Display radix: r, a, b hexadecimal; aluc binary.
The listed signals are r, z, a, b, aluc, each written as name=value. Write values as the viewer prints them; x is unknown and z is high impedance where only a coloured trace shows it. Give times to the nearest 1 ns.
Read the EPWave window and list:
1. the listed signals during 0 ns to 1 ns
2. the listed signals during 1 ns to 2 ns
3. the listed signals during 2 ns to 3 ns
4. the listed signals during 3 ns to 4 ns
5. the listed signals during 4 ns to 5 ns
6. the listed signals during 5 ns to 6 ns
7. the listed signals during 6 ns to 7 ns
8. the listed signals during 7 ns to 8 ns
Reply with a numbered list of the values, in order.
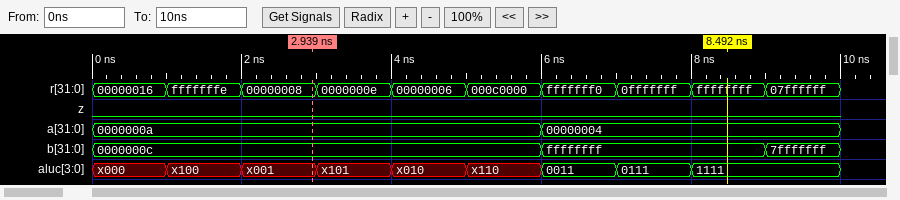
1. r=00000016, z=0, a=0000000a, b=0000000c, aluc=x000
2. r=fffffffe, z=0, a=0000000a, b=0000000c, aluc=x100
3. r=00000008, z=0, a=0000000a, b=0000000c, aluc=x001
4. r=0000000e, z=0, a=0000000a, b=0000000c, aluc=x101
5. r=00000006, z=0, a=0000000a, b=0000000c, aluc=x010
6. r=000c0000, z=0, a=0000000a, b=0000000c, aluc=x110
7. r=fffffff0, z=0, a=00000004, b=ffffffff, aluc=0011
8. r=0fffffff, z=0, a=00000004, b=ffffffff, aluc=0111
